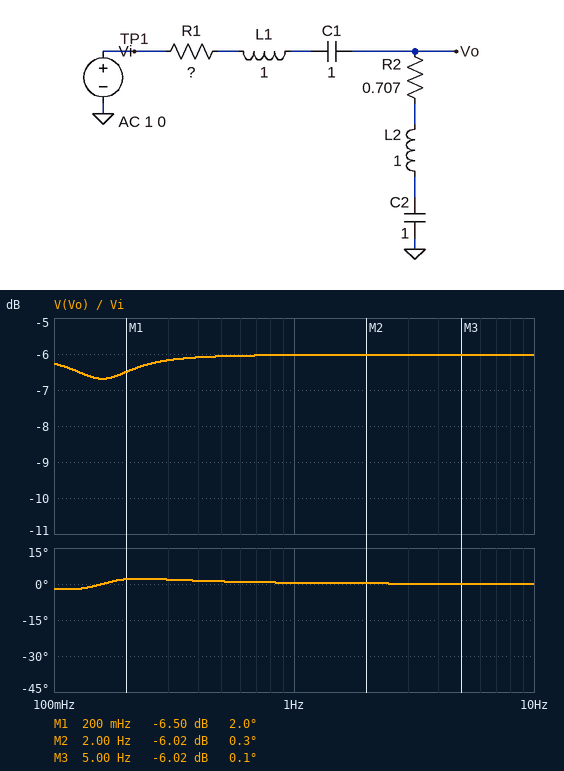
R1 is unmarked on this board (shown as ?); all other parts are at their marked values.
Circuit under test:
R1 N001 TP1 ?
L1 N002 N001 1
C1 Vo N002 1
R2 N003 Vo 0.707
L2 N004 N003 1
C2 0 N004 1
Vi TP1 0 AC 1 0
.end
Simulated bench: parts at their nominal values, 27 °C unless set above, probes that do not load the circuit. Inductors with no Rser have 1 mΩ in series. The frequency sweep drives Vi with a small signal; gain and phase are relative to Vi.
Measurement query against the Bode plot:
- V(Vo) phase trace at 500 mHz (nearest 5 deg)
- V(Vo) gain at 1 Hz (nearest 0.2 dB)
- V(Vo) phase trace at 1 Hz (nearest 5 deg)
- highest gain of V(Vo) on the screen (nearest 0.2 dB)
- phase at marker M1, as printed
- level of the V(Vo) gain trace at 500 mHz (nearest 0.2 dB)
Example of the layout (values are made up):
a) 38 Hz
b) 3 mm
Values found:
a) 0 deg
b) -6.0 dB
c) 0 deg
d) -6.0 dB
e) 2.0 deg
f) -6.0 dB
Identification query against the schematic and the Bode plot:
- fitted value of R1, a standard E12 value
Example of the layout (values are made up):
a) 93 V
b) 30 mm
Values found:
a) 0.82 Ω
